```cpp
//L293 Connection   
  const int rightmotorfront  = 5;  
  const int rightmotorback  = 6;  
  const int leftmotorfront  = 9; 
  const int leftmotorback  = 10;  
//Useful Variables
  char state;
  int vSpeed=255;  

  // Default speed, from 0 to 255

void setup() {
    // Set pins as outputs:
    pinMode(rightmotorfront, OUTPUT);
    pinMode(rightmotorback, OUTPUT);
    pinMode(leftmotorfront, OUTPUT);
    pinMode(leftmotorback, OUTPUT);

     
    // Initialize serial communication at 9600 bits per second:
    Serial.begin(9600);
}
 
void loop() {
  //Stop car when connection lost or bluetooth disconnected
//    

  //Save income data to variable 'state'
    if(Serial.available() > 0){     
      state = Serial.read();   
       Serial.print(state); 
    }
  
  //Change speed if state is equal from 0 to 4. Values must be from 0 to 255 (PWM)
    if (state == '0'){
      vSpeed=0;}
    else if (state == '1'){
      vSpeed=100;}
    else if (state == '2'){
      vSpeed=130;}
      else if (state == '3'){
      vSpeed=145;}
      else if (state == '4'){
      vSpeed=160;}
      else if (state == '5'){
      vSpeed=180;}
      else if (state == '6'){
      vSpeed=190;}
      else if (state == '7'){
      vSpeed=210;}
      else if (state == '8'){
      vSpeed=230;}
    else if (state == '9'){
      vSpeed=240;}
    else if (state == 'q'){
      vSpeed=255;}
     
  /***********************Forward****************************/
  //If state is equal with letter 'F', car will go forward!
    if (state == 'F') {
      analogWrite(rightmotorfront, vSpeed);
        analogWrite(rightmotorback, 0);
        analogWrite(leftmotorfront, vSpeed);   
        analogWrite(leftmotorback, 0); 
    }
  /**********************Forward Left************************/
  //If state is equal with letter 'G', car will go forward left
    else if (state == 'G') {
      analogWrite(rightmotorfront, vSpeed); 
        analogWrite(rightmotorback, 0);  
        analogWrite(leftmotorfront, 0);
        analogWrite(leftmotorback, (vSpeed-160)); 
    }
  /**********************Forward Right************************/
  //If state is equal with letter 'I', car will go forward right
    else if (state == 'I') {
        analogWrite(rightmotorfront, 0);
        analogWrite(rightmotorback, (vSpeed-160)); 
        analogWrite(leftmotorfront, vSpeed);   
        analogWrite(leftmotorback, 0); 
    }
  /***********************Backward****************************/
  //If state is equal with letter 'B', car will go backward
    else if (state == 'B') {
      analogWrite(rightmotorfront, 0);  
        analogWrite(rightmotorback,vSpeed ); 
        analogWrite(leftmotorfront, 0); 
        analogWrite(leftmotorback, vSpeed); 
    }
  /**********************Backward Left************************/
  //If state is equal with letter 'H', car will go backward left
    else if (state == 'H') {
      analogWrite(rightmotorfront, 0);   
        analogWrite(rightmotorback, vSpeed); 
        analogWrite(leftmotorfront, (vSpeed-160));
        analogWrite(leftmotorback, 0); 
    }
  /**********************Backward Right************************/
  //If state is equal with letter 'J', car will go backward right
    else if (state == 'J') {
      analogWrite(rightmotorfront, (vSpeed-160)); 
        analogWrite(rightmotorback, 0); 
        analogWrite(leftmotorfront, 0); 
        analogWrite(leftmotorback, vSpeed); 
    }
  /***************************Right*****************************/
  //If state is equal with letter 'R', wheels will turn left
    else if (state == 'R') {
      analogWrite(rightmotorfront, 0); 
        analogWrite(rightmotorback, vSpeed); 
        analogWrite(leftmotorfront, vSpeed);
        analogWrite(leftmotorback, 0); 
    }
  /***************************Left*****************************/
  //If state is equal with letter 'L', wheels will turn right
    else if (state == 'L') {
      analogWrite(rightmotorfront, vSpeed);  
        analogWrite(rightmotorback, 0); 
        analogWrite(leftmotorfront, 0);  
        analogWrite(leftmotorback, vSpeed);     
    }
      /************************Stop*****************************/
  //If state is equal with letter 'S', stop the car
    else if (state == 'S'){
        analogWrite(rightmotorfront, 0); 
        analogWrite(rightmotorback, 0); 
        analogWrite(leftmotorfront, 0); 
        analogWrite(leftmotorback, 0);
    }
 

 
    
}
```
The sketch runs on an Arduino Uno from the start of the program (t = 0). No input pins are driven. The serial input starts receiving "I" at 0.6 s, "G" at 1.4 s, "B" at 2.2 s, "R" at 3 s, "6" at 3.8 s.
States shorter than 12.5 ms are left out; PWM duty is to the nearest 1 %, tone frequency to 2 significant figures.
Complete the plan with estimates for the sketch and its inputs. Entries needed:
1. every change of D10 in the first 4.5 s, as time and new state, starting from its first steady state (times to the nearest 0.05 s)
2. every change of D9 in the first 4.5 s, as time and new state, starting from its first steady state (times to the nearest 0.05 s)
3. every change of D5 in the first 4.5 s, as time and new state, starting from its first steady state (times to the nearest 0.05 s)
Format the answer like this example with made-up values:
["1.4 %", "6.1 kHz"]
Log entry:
["0 s low; 1.4 s PWM 37 %; 2.2 s high; 3 s low", "0 s low; 0.6 s high; 1.4 s low; 3 s high", "0 s low; 1.4 s high; 2.2 s low"]
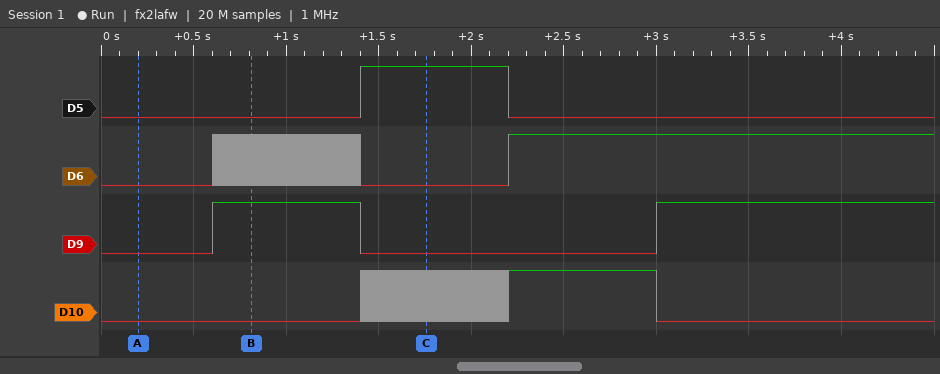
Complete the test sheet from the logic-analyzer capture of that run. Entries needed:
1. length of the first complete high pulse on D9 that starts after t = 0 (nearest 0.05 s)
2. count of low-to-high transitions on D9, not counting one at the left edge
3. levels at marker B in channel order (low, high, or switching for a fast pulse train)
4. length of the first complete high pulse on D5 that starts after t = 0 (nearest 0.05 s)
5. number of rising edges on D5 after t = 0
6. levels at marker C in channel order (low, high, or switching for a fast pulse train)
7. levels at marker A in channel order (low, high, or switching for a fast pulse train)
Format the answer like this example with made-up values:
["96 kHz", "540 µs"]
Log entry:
["0.80 s", "2", "D5 low, D6 switching, D9 high, D10 low", "0.80 s", "1", "D5 high, D6 low, D9 low, D10 switching", "D5 low, D6 low, D9 low, D10 low"]
